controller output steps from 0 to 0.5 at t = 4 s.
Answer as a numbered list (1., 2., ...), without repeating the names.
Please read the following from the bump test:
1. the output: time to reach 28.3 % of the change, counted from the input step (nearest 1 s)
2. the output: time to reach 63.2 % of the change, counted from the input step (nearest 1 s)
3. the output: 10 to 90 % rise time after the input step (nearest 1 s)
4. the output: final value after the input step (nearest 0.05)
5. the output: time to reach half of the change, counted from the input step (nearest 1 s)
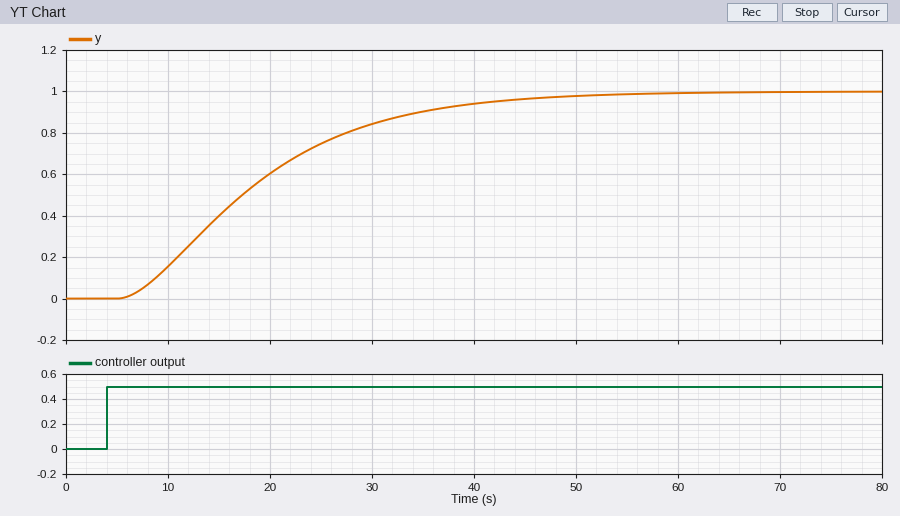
1. 9 s
2. 17 s
3. 26 s
4. 1.00
5. 13 s
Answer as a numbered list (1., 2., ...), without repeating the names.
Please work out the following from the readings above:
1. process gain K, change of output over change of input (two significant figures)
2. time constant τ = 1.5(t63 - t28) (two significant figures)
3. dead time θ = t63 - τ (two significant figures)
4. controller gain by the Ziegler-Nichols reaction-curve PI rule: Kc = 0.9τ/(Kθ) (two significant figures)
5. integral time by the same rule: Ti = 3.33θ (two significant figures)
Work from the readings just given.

1. 2.0
2. 12 s
3. 5.0 s
4. 1.1
5. 17 s
